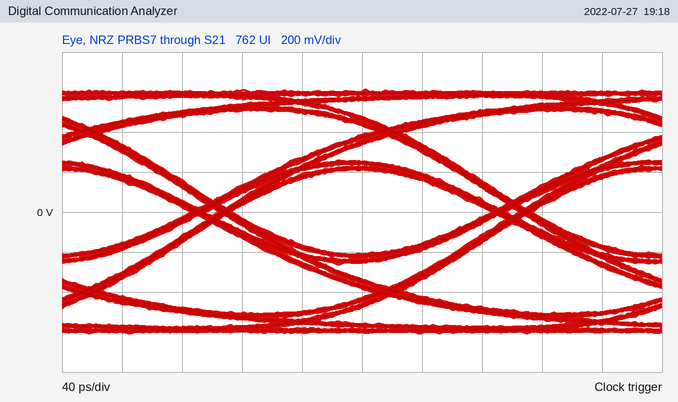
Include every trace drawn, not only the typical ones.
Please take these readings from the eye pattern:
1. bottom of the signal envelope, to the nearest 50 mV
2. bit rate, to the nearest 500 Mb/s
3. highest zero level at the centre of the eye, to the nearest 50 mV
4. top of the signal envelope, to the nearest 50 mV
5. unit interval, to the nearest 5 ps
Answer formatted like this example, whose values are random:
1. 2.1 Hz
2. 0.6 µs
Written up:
1. -600 mV
2. 5.0 Gb/s
3. -200 mV
4. 600 mV
5. 200 ps
